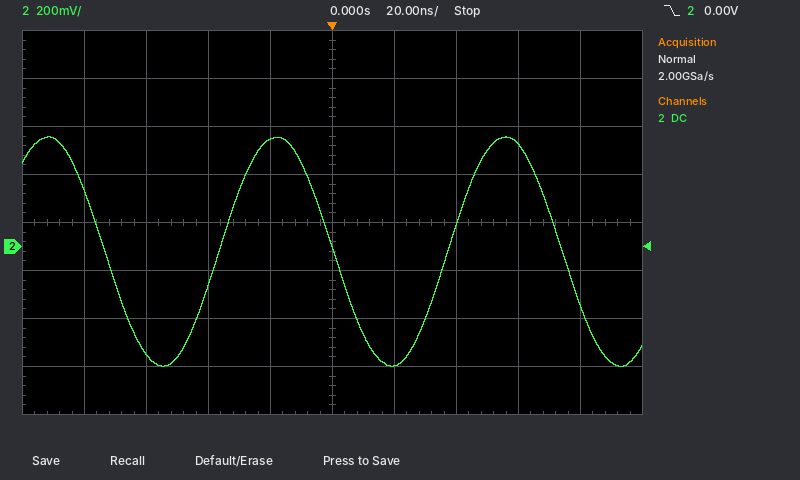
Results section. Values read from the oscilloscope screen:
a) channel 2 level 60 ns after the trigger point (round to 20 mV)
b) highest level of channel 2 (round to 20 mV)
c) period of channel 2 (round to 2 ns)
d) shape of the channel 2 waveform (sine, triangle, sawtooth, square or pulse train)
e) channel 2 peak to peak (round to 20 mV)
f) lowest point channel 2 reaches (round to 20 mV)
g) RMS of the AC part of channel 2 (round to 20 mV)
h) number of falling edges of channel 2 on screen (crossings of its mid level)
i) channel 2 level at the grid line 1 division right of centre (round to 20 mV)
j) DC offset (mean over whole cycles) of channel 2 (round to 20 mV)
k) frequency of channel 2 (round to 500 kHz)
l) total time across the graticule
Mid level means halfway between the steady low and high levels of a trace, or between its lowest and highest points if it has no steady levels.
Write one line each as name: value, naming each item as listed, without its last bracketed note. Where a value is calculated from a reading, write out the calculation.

channel 2 level 60 ns after the trigger point: 420 mV
highest level of channel 2: 460 mV
period of channel 2: 74 ns
shape of the channel 2 waveform: sine
channel 2 peak to peak: 460 mV − (-500 mV) = 960 mV
lowest point channel 2 reaches: -500 mV
RMS of the AC part of channel 2: 960 mV / (2√2) ≈ 339 mV, so 340 mV to the nearest 20 mV
number of falling edges of channel 2 on screen: 3
channel 2 level at the grid line 1 division right of centre: -500 mV
DC offset (mean over whole cycles) of channel 2: (460 mV + (-500 mV)) / 2 ≈ -20 mV
frequency of channel 2: 1 / 74 ns ≈ 13.5 MHz
total time across the graticule: 200 ns
